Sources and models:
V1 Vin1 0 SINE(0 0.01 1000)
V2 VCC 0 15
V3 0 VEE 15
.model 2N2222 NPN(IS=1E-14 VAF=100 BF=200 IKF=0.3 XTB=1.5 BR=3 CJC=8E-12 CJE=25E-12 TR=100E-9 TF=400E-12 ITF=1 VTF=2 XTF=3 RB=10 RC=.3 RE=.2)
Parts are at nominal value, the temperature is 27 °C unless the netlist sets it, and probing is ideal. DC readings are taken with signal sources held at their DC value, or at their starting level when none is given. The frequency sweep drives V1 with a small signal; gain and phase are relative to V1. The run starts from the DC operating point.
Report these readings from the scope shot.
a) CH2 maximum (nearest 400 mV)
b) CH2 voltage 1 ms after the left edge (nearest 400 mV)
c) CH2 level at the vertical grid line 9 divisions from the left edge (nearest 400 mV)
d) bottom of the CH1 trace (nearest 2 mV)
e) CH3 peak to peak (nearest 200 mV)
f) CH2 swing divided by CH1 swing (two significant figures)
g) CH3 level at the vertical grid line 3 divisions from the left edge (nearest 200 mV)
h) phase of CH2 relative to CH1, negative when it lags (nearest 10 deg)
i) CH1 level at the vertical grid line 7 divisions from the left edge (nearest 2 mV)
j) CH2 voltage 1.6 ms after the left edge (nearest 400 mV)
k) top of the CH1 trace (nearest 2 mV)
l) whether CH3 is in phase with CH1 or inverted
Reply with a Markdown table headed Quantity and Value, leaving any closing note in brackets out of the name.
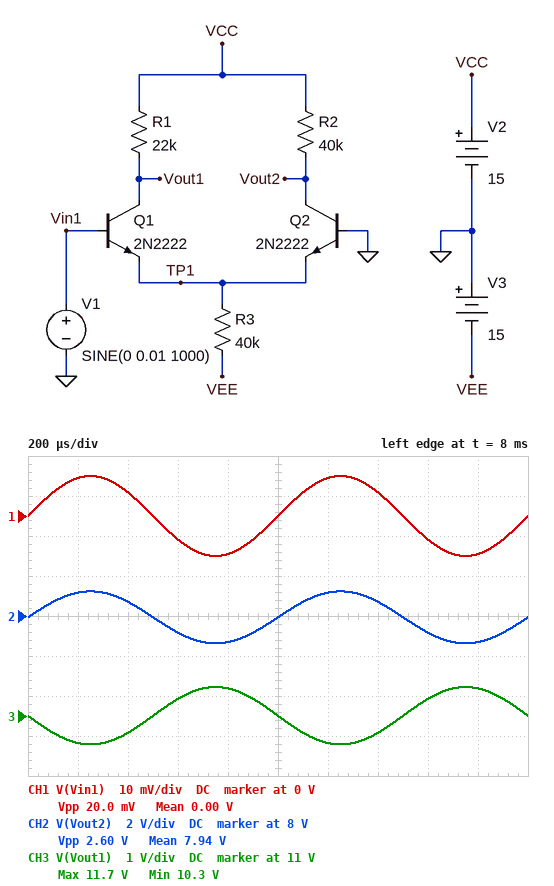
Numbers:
| Quantity | Value |
|---|---|
| CH2 maximum | 9.2 V |
| CH2 voltage 1 ms after the left edge | 8.0 V |
| CH2 level at the vertical grid line 9 divisions from the left edge | 6.8 V |
| bottom of the CH1 trace | -10 mV |
| CH3 peak to peak | 1.4 V |
| CH2 swing divided by CH1 swing | 130 |
| CH3 level at the vertical grid line 3 divisions from the left edge | 11.4 V |
| phase of CH2 relative to CH1, negative when it lags | 0 deg |
| CH1 level at the vertical grid line 7 divisions from the left edge | 6 mV |
| CH2 voltage 1.6 ms after the left edge | 7.2 V |
| top of the CH1 trace | 10 mV |
| whether CH3 is in phase with CH1 or inverted | inverted |
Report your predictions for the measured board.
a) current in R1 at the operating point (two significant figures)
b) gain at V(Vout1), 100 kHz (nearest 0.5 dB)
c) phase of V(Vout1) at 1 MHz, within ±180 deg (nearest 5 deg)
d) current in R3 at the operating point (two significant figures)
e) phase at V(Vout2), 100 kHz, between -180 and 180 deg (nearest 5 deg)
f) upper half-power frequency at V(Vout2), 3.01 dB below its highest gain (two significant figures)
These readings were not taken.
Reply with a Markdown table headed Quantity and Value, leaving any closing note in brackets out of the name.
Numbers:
| Quantity | Value |
|---|---|
| current in R1 at the operating point | 180 µA |
| gain at V(Vout1), 100 kHz | 37.0 dB |
| phase of V(Vout1) at 1 MHz, within ±180 deg | 155 deg |
| current in R3 at the operating point | 360 µA |
| phase at V(Vout2), 100 kHz, between -180 and 180 deg | -5 deg |
| upper half-power frequency at V(Vout2), 3.01 dB below its highest gain | 1.1 MHz |
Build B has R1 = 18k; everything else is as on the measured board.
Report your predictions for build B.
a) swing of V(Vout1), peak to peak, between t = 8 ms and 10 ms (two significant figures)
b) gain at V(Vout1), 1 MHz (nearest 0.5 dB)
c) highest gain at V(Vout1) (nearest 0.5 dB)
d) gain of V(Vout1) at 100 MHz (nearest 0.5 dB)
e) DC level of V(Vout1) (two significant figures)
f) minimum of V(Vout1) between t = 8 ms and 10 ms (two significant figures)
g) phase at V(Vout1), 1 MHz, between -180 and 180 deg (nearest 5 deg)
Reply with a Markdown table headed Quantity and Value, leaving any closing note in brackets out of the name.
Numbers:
| Quantity | Value |
|---|---|
| swing of V(Vout1), peak to peak, between t = 8 ms and 10 ms | 1.2 V |
| gain at V(Vout1), 1 MHz | 35.0 dB |
| highest gain at V(Vout1) | 35.5 dB |
| gain of V(Vout1) at 100 MHz | 6.0 dB |
| DC level of V(Vout1) | 12 V |
| minimum of V(Vout1) between t = 8 ms and 10 ms | 11 V |
| phase at V(Vout1), 1 MHz, between -180 and 180 deg | 160 deg |
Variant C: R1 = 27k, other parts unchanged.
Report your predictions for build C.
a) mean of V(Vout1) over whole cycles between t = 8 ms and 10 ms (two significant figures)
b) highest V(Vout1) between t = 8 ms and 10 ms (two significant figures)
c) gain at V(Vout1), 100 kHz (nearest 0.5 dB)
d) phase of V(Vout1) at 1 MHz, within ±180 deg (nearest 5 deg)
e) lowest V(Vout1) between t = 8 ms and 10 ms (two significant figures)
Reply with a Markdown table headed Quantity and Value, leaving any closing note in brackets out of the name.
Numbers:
| Quantity | Value |
|---|---|
| mean of V(Vout1) over whole cycles between t = 8 ms and 10 ms | 10 V |
| highest V(Vout1) between t = 8 ms and 10 ms | 11 V |
| gain at V(Vout1), 100 kHz | 39.0 dB |
| phase of V(Vout1) at 1 MHz, within ±180 deg | 150 deg |
| lowest V(Vout1) between t = 8 ms and 10 ms | 9.2 V |
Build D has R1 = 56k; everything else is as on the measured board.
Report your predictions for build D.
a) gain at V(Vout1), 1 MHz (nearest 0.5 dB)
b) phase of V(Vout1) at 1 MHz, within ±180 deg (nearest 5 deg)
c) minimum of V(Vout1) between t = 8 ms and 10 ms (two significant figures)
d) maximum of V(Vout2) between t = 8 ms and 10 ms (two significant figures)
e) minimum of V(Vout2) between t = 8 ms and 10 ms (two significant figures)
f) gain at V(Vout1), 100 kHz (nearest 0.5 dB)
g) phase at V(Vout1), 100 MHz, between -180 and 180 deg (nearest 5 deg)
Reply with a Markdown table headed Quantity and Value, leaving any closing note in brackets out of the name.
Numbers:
| Quantity | Value |
|---|---|
| gain at V(Vout1), 1 MHz | 40.5 dB |
| phase of V(Vout1) at 1 MHz, within ±180 deg | 125 deg |
| minimum of V(Vout1) between t = 8 ms and 10 ms | 3.3 V |
| maximum of V(Vout2) between t = 8 ms and 10 ms | 9.0 V |
| minimum of V(Vout2) between t = 8 ms and 10 ms | 6.5 V |
| gain at V(Vout1), 100 kHz | 45.0 dB |
| phase at V(Vout1), 100 MHz, between -180 and 180 deg | 40 deg |
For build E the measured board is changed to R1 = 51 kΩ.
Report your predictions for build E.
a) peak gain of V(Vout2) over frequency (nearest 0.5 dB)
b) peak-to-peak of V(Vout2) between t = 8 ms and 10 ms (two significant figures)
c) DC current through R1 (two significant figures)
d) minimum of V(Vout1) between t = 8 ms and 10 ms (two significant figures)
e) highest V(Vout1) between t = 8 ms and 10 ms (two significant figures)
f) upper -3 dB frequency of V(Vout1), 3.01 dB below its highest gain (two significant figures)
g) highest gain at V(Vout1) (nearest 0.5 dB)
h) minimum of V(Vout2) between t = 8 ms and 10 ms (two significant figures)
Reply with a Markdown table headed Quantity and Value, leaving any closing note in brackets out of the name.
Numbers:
| Quantity | Value |
|---|---|
| peak gain of V(Vout2) over frequency | 42.0 dB |
| peak-to-peak of V(Vout2) between t = 8 ms and 10 ms | 2.5 V |
| DC current through R1 | 180 µA |
| minimum of V(Vout1) between t = 8 ms and 10 ms | 4.3 V |
| highest V(Vout1) between t = 8 ms and 10 ms | 7.6 V |
| upper -3 dB frequency of V(Vout1), 3.01 dB below its highest gain | 810 kHz |
| highest gain at V(Vout1) | 44.5 dB |
| minimum of V(Vout2) between t = 8 ms and 10 ms | 6.5 V |
